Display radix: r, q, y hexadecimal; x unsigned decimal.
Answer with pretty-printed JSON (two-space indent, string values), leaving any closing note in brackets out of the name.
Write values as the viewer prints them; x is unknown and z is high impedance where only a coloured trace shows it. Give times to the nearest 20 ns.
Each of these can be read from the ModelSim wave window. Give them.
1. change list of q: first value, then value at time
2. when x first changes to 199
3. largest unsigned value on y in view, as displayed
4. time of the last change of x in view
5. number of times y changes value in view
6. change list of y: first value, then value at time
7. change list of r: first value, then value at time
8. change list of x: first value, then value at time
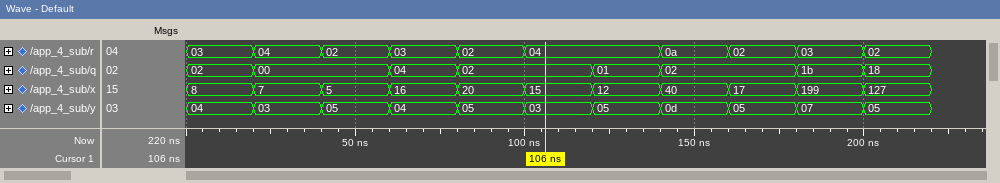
{
  "change list of q: first value, then value at time": "02, 00 at 20 ns, 04 at 60 ns, 02 at 80 ns, 01 at 120 ns, 02 at 140 ns, 1b at 180 ns, 18 at 200 ns",
  "when x first changes to 199": "180 ns",
  "largest unsigned value on y in view, as displayed": "0d",
  "time of the last change of x in view": "200 ns",
  "number of times y changes value in view": "10",
  "change list of y: first value, then value at time": "04, 03 at 20 ns, 05 at 40 ns, 04 at 60 ns, 05 at 80 ns, 03 at 100 ns, 05 at 120 ns, 0d at 140 ns, 05 at 160 ns, 07 at 180 ns, 05 at 200 ns",
  "change list of r: first value, then value at time": "03, 04 at 20 ns, 02 at 40 ns, 03 at 60 ns, 02 at 80 ns, 04 at 100 ns, 0a at 140 ns, 02 at 160 ns, 03 at 180 ns, 02 at 200 ns",
  "change list of x: first value, then value at time": "8, 7 at 20 ns, 5 at 40 ns, 16 at 60 ns, 20 at 80 ns, 15 at 100 ns, 12 at 120 ns, 40 at 140 ns, 17 at 160 ns, 199 at 180 ns, 127 at 200 ns"
}
